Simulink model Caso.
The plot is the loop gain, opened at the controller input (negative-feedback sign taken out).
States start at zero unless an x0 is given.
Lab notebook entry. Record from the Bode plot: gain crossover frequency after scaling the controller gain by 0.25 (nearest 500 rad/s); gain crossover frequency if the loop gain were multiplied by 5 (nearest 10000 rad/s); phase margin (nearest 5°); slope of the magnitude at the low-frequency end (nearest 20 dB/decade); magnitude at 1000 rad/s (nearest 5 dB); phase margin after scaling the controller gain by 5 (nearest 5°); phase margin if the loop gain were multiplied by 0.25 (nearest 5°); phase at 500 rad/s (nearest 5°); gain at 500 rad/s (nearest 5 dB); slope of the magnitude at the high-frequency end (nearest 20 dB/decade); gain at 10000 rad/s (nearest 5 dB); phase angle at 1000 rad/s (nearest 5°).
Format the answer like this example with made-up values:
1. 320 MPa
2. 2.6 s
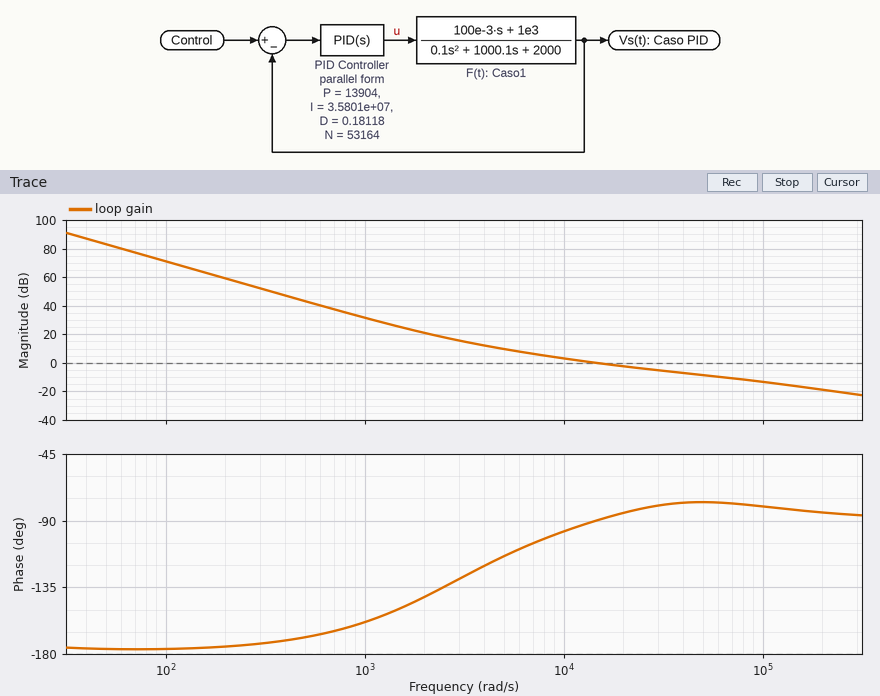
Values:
1. 4000 rad/s
2. 110000 rad/s
3. 90°
4. -40 dB/decade
5. 30 dB
6. 100°
7. 60°
8. -170°
9. 45 dB
10. -20 dB/decade
11. 5 dB
12. -160°
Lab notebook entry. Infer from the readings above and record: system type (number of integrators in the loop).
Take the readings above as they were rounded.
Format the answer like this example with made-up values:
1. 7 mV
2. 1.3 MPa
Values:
1. 2
